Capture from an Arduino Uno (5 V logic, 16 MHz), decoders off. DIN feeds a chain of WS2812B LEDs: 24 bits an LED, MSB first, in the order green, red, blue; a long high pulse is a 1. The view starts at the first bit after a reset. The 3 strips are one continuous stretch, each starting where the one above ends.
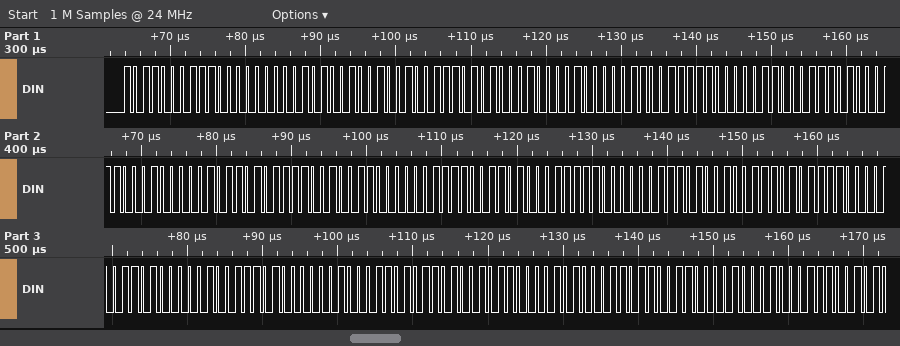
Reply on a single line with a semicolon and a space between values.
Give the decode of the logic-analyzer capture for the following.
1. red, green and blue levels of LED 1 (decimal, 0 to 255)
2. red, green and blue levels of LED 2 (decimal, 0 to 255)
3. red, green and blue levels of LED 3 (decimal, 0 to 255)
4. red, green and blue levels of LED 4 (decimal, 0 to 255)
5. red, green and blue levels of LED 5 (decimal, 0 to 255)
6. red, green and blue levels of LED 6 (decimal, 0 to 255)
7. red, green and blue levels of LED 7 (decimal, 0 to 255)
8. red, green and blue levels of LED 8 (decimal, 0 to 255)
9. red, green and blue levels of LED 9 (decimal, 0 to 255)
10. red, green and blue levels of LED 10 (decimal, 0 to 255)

192, 177, 20; 117, 146, 16; 62, 131, 12; 98, 116, 11; 76, 94, 15; 124, 52, 14; 175, 147, 3; 58, 65, 4; 75, 107, 10; 97, 54, 17
